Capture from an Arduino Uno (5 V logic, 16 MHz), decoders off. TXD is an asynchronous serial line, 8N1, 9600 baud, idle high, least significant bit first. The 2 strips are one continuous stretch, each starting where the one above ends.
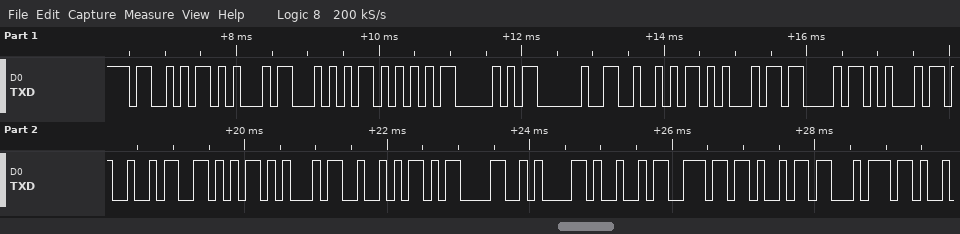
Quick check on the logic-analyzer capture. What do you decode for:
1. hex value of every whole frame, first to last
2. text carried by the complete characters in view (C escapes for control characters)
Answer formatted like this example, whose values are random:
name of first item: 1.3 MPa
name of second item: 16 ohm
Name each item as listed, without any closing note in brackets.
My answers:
hex value of every whole frame, first to last: 53 45 54 55 50 20 52 45 43 45 49 56 45 52 0D 0A 49 6E 69 74
text carried by the complete characters in view: "SETUP RECEIVER\r\nInit"
